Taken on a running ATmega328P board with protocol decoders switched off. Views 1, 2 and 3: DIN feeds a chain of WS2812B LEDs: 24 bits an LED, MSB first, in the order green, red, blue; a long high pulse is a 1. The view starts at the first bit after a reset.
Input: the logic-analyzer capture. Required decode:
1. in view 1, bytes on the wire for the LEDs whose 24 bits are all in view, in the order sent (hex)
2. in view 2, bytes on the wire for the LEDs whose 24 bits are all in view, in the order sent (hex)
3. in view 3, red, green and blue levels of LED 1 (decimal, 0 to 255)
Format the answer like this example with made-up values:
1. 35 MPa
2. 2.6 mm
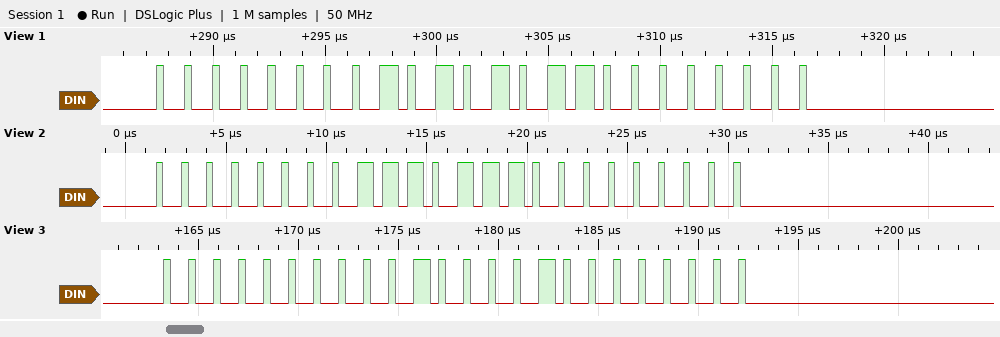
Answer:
1. 00 AB 00
2. 00 EE 00
3. 33, 0, 0
